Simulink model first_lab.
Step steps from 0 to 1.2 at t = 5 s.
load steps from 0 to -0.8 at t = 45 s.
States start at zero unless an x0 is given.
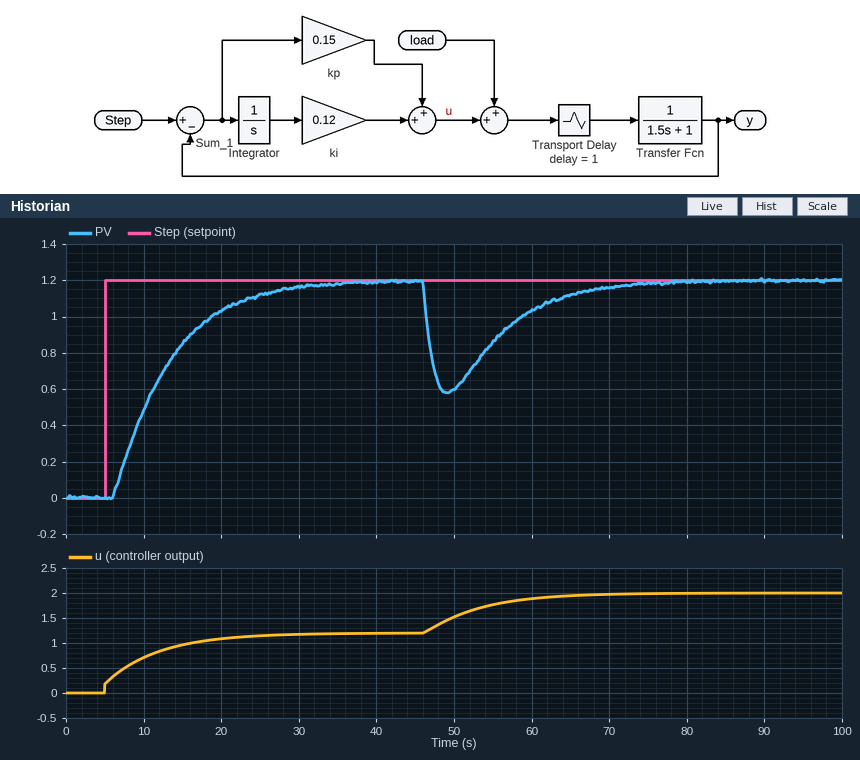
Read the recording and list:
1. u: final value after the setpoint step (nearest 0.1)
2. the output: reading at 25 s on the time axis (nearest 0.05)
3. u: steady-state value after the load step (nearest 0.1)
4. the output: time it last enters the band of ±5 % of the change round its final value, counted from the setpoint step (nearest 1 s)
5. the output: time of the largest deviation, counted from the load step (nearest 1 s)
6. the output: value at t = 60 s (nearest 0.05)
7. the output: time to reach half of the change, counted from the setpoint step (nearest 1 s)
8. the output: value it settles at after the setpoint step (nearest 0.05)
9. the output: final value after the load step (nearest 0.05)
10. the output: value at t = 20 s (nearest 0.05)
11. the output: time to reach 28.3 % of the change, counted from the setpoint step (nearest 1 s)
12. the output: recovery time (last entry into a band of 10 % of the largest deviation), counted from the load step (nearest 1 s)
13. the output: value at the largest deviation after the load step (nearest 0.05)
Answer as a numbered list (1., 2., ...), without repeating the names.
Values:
1. 1.2
2. 1.10
3. 2.0
4. 22 s
5. 4 s
6. 1.05
7. 6 s
8. 1.20
9. 1.20
10. 1.05
11. 4 s
12. 22 s
13. 0.60
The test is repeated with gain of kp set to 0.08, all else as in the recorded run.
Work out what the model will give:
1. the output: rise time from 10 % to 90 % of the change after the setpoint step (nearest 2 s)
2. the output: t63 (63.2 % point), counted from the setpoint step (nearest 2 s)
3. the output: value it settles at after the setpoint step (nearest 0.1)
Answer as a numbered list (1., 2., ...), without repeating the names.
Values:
1. 14 s
2. 8 s
3. 1.2
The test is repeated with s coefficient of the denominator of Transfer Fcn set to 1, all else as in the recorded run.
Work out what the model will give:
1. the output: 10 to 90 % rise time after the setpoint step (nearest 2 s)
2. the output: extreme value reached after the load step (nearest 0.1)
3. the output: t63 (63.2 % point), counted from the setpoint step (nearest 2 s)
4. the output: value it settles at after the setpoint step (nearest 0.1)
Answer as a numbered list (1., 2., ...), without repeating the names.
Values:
1. 16 s
2. 0.5
3. 8 s
4. 1.2
